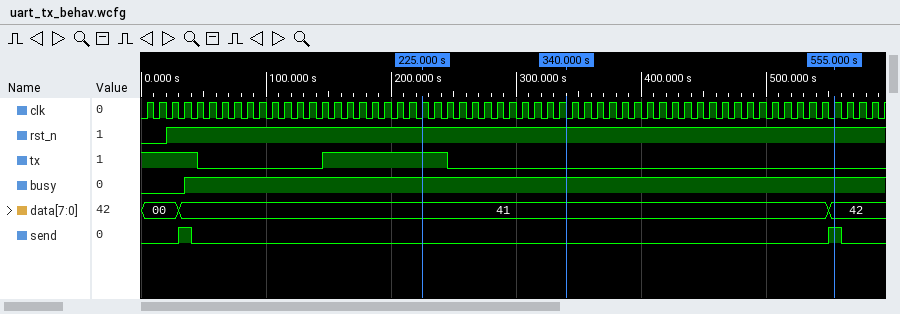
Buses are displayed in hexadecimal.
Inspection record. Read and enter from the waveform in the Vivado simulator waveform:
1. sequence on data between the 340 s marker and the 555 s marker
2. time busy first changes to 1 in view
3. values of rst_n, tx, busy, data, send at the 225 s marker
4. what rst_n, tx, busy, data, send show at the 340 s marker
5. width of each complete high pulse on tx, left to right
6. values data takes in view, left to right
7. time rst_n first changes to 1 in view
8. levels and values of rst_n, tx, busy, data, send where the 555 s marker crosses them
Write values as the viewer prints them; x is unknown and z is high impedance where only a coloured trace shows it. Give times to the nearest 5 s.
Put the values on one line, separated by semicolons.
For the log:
41, 42; 35 s; rst_n=1, tx=1, busy=1, data=41, send=0; rst_n=1, tx=0, busy=1, data=41, send=0; 100 s; 00, 41, 42; 20 s; rst_n=1, tx=0, busy=1, data=42, send=1
